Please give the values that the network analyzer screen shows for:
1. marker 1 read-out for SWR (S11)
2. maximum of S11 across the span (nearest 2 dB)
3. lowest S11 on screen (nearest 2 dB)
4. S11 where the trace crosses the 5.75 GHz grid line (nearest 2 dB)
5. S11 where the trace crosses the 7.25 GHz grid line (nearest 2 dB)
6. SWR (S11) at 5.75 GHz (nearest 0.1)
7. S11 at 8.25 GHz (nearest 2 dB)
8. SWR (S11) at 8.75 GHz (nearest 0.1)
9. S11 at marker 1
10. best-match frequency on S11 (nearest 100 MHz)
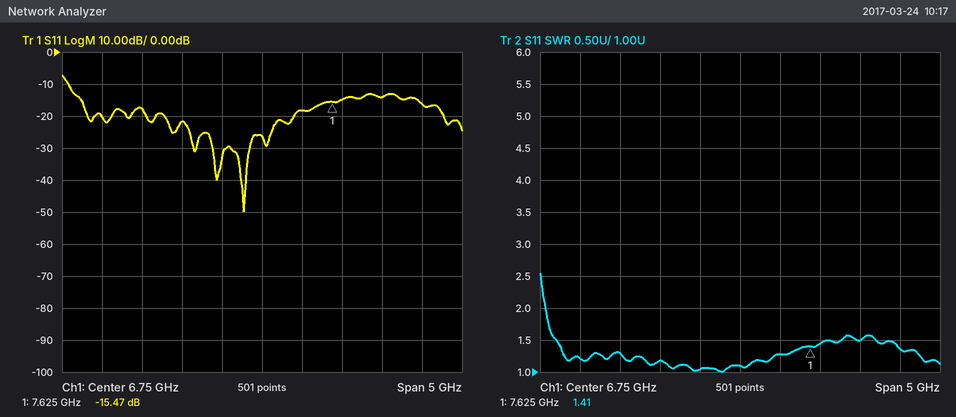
1.41
-8 dB
-50 dB
-22 dB
-18 dB
1.2
-14 dB
1.4
-15.47 dB
6.5 GHz
